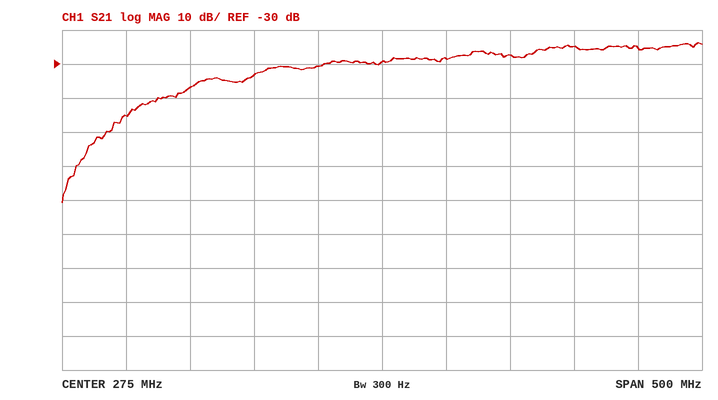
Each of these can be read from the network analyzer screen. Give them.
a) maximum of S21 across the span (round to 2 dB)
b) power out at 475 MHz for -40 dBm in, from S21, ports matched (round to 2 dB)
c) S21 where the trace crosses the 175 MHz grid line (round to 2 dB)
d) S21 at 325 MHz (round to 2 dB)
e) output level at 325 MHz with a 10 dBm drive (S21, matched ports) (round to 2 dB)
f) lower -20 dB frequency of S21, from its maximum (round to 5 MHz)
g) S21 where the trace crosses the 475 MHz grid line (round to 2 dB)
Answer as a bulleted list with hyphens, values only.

- -24 dB
- -66 dBm
- -34 dB
- -28 dB
- -18 dBm
- 80 MHz
- -26 dB
